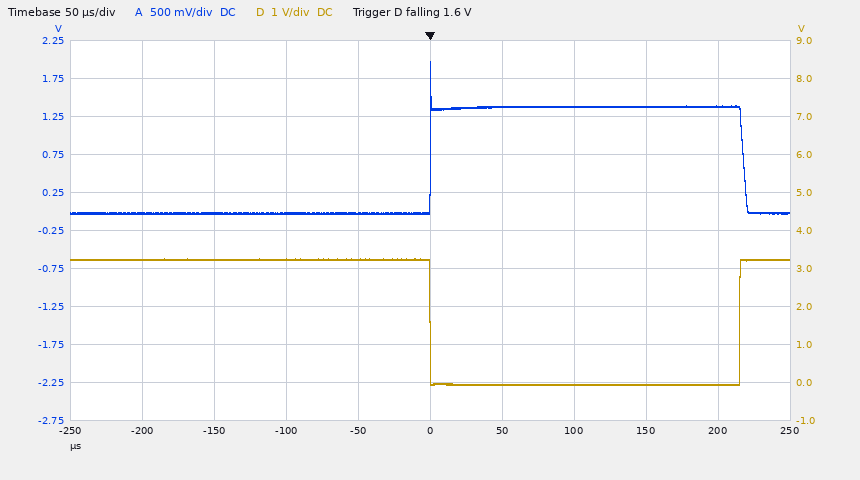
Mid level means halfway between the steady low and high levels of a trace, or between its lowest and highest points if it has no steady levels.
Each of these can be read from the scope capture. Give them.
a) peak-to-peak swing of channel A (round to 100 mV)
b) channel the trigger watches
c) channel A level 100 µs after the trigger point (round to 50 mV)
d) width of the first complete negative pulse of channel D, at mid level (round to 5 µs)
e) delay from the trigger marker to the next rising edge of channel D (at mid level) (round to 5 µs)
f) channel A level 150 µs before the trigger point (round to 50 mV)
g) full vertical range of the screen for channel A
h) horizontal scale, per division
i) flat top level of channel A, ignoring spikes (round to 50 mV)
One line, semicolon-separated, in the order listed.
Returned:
2.00 V; channel D; 1.40 V; 215 µs; 215 µs; 0 mV; 5 V; 50 µs; 1.40 V
